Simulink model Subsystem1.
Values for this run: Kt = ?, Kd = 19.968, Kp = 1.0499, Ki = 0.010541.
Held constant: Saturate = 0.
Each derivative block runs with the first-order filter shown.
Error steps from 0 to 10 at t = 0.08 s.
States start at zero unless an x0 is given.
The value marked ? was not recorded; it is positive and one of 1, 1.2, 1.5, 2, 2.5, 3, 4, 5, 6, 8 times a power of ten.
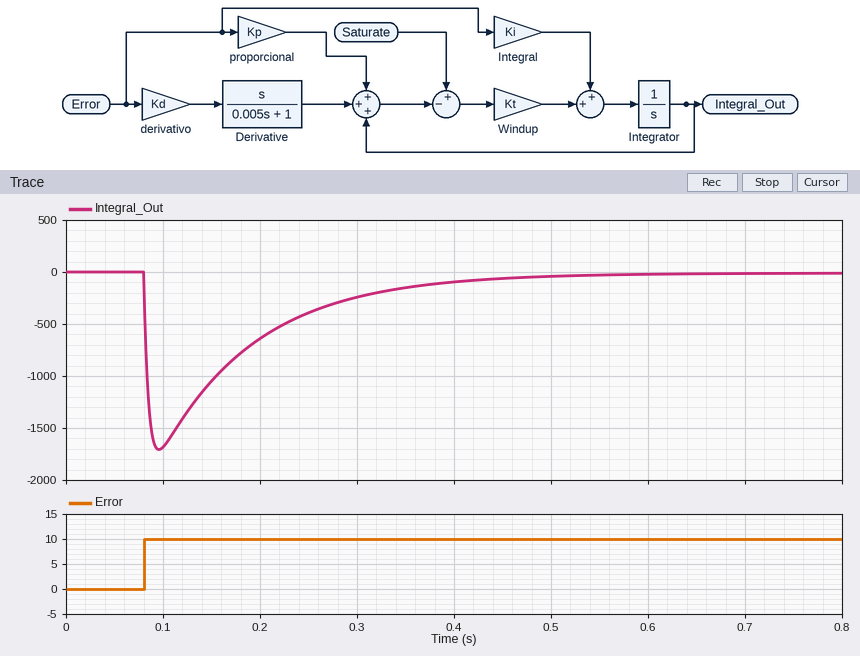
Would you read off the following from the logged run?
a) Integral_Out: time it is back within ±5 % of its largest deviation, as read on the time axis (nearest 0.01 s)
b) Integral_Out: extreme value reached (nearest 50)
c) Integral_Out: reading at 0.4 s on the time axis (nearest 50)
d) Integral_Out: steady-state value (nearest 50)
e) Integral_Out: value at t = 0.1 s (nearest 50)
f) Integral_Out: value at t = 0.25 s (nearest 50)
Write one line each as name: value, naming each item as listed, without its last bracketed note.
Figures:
Integral_Out: time it is back within ±5 % of its largest deviation, as read on the time axis: 0.40 s
Integral_Out: extreme value reached: -1700
Integral_Out: reading at 0.4 s on the time axis: -100
Integral_Out: steady-state value: 0
Integral_Out: value at t = 0.1 s: -1700
Integral_Out: value at t = 0.25 s: -400
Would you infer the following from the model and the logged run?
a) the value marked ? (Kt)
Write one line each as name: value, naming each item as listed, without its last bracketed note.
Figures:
the value marked ?: 10
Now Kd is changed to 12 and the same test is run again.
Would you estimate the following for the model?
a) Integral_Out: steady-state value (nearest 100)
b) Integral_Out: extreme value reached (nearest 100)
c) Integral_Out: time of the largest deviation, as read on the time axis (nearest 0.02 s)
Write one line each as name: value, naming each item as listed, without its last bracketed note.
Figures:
Integral_Out: steady-state value: 0
Integral_Out: extreme value reached: -1000
Integral_Out: time of the largest deviation, as read on the time axis: 0.10 s
